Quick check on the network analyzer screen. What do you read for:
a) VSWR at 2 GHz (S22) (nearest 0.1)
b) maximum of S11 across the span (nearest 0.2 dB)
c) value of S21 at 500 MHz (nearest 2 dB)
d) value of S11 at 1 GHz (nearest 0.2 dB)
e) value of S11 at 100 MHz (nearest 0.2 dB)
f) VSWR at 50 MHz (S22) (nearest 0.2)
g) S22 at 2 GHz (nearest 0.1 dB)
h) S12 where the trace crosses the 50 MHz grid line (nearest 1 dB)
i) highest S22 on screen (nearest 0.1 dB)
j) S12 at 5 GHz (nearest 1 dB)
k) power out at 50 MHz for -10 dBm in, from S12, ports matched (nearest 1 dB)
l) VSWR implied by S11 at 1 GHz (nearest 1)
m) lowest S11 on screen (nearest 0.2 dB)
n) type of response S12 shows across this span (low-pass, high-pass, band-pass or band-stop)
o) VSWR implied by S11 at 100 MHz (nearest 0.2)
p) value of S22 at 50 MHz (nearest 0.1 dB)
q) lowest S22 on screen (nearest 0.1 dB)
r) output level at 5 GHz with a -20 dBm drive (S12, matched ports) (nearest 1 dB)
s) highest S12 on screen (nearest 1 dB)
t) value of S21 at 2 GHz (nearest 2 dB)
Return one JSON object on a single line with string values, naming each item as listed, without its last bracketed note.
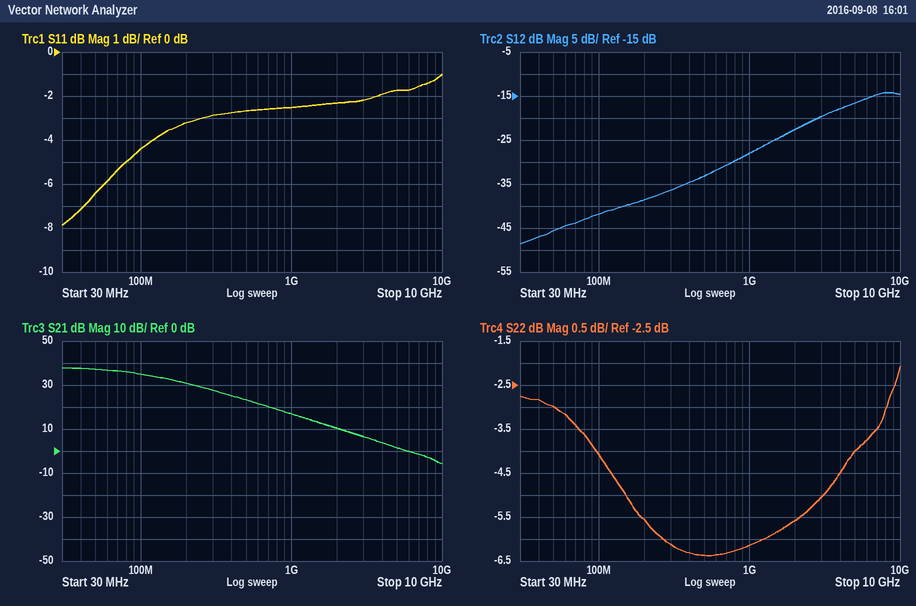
{"VSWR at 2 GHz (S22)": "3.2", "maximum of S11 across the span": "-1.0 dB", "value of S21 at 500 MHz": "24 dB", "value of S11 at 1 GHz": "-2.6 dB", "value of S11 at 100 MHz": "-4.4 dB", "VSWR at 50 MHz (S22)": "5.8", "S22 at 2 GHz": "-5.6 dB", "S12 where the trace crosses the 50 MHz grid line": "-46 dB", "highest S22 on screen": "-2.1 dB", "S12 at 5 GHz": "-17 dB", "power out at 50 MHz for -10 dBm in, from S12, ports matched": "-56 dBm", "VSWR implied by S11 at 1 GHz": "7", "lowest S11 on screen": "-7.8 dB", "type of response S12 shows across this span": "high-pass", "VSWR implied by S11 at 100 MHz": "4.0", "value of S22 at 50 MHz": "-3.0 dB", "lowest S22 on screen": "-6.4 dB", "output level at 5 GHz with a -20 dBm drive (S12, matched ports)": "-37 dBm", "highest S12 on screen": "-14 dB", "value of S21 at 2 GHz": "10 dB"}
